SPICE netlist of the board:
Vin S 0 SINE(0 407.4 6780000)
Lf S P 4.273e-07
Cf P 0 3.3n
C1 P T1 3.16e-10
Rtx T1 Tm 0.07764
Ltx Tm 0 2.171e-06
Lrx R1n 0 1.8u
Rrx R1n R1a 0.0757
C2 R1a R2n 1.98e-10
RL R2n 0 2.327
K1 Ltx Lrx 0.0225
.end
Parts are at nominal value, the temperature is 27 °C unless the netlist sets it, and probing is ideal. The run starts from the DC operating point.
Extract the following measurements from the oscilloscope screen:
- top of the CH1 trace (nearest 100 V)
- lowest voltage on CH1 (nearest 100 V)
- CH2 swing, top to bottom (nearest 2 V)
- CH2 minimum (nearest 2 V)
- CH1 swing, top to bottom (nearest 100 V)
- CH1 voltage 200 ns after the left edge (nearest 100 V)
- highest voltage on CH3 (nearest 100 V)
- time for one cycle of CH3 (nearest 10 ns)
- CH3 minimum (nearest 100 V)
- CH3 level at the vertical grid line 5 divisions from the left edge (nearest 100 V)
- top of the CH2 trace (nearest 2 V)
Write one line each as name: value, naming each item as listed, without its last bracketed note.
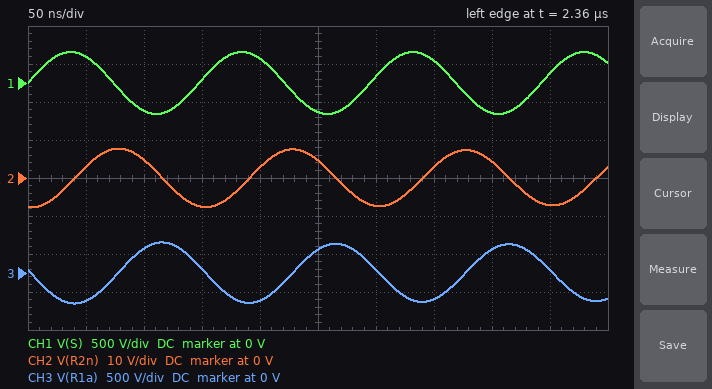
top of the CH1 trace: 400 V
lowest voltage on CH1: -400 V
CH2 swing, top to bottom: 16 V
CH2 minimum: -8 V
CH1 swing, top to bottom: 800 V
CH1 voltage 200 ns after the left edge: 300 V
highest voltage on CH3: 400 V
time for one cycle of CH3: 150 ns
CH3 minimum: -400 V
CH3 level at the vertical grid line 5 divisions from the left edge: 300 V
top of the CH2 trace: 8 V
